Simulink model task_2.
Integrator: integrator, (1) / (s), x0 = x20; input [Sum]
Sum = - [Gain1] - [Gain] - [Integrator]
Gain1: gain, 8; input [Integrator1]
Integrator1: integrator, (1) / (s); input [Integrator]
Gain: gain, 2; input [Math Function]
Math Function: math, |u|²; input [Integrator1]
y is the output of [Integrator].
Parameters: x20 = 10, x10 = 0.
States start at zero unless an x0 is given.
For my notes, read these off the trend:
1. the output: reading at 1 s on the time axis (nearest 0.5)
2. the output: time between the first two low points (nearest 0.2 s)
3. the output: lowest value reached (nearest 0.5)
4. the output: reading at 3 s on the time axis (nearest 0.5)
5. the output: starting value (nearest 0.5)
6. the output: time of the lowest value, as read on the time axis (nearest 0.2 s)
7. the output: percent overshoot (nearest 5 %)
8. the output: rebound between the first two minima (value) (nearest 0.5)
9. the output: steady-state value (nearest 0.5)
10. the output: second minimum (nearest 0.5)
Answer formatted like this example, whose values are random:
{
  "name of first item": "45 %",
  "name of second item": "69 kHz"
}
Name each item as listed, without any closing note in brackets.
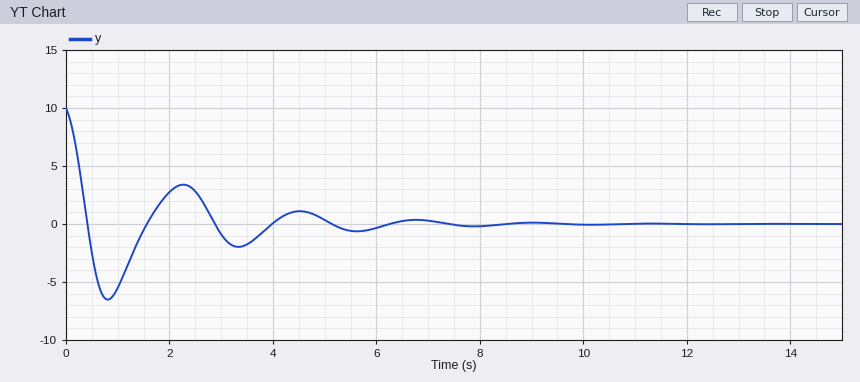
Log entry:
{
  "the output: reading at 1 s on the time axis": "-5.5",
  "the output: time between the first two low points": "2.6 s",
  "the output: lowest value reached": "-6.5",
  "the output: reading at 3 s on the time axis": "-1.0",
  "the output: starting value": "10.0",
  "the output: time of the lowest value, as read on the time axis": "0.8 s",
  "the output: percent overshoot": "65 %",
  "the output: rebound between the first two minima (value)": "3.5",
  "the output: steady-state value": "0.0",
  "the output: second minimum": "-2.0"
}
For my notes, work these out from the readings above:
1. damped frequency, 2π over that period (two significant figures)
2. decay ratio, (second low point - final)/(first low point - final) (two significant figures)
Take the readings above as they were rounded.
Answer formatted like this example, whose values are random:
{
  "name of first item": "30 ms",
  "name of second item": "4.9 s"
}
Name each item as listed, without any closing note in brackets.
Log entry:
{
  "damped frequency, 2π over that period": "2.4 rad/s",
  "decay ratio, (second low point - final)/(first low point - final)": "0.31"
}
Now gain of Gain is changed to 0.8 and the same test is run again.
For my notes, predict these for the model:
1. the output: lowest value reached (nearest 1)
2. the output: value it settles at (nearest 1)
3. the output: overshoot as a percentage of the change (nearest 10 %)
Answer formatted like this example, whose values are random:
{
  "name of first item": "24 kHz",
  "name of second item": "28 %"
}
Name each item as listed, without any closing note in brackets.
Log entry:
{
  "the output: lowest value reached": "-6",
  "the output: value it settles at": "0",
  "the output: overshoot as a percentage of the change": "60 %"
}
